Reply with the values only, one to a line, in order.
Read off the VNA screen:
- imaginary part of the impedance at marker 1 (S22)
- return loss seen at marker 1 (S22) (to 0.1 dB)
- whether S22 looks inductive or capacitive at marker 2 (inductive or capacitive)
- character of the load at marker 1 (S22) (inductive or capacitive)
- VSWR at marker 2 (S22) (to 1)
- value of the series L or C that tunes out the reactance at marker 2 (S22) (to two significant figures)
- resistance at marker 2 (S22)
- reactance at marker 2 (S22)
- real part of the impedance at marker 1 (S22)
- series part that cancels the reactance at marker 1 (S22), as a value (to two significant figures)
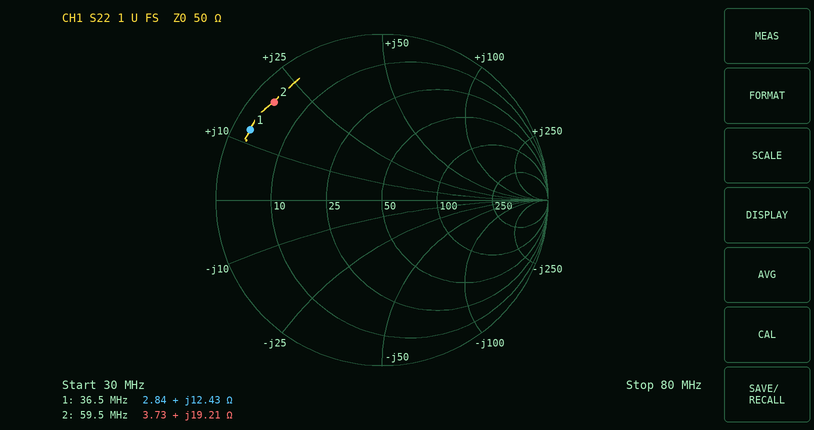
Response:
+12.43 Ω
0.9 dB
inductive
inductive
15
140 pF
3.73 Ω
+19.21 Ω
2.84 Ω
350 pF
